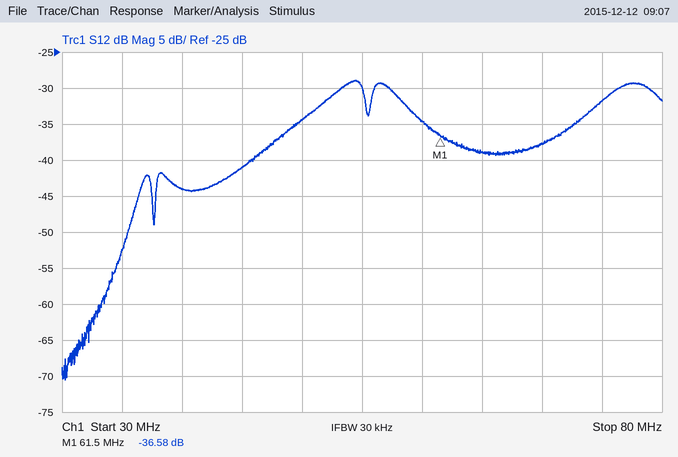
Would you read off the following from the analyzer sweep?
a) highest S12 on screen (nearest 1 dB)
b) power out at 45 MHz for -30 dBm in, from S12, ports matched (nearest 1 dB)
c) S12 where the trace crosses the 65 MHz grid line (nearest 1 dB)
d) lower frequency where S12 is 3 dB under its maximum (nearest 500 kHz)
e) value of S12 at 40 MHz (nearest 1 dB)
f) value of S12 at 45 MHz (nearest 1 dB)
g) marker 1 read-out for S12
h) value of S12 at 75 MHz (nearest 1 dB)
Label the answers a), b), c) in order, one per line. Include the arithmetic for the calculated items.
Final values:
a) -29 dB
b) -30 dBm + (-41 dB) = -71 dBm
c) -39 dB
d) 52.0 MHz
e) -44 dB
f) -41 dB
g) -36.58 dB
h) -32 dB
